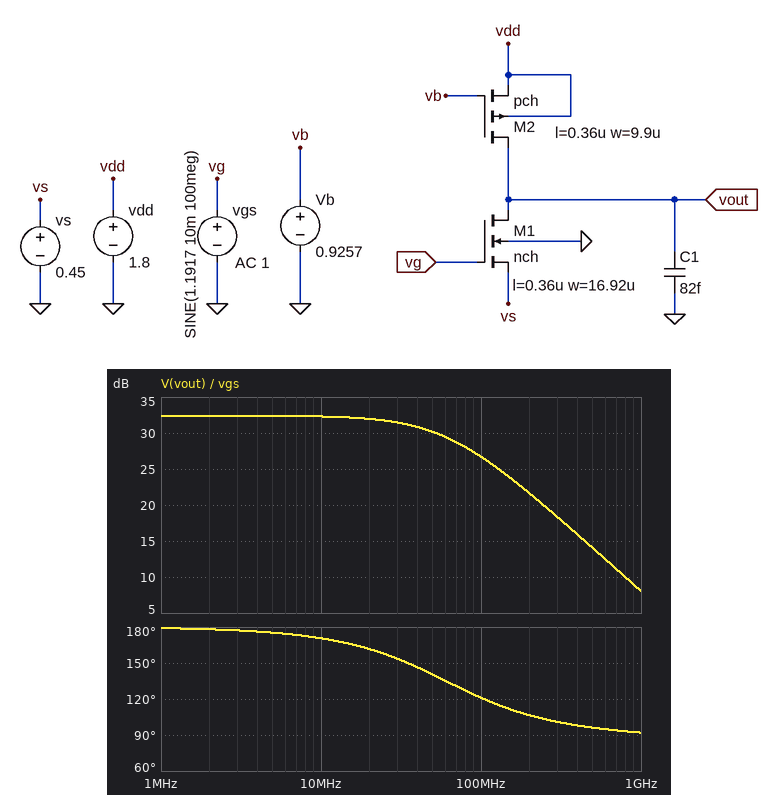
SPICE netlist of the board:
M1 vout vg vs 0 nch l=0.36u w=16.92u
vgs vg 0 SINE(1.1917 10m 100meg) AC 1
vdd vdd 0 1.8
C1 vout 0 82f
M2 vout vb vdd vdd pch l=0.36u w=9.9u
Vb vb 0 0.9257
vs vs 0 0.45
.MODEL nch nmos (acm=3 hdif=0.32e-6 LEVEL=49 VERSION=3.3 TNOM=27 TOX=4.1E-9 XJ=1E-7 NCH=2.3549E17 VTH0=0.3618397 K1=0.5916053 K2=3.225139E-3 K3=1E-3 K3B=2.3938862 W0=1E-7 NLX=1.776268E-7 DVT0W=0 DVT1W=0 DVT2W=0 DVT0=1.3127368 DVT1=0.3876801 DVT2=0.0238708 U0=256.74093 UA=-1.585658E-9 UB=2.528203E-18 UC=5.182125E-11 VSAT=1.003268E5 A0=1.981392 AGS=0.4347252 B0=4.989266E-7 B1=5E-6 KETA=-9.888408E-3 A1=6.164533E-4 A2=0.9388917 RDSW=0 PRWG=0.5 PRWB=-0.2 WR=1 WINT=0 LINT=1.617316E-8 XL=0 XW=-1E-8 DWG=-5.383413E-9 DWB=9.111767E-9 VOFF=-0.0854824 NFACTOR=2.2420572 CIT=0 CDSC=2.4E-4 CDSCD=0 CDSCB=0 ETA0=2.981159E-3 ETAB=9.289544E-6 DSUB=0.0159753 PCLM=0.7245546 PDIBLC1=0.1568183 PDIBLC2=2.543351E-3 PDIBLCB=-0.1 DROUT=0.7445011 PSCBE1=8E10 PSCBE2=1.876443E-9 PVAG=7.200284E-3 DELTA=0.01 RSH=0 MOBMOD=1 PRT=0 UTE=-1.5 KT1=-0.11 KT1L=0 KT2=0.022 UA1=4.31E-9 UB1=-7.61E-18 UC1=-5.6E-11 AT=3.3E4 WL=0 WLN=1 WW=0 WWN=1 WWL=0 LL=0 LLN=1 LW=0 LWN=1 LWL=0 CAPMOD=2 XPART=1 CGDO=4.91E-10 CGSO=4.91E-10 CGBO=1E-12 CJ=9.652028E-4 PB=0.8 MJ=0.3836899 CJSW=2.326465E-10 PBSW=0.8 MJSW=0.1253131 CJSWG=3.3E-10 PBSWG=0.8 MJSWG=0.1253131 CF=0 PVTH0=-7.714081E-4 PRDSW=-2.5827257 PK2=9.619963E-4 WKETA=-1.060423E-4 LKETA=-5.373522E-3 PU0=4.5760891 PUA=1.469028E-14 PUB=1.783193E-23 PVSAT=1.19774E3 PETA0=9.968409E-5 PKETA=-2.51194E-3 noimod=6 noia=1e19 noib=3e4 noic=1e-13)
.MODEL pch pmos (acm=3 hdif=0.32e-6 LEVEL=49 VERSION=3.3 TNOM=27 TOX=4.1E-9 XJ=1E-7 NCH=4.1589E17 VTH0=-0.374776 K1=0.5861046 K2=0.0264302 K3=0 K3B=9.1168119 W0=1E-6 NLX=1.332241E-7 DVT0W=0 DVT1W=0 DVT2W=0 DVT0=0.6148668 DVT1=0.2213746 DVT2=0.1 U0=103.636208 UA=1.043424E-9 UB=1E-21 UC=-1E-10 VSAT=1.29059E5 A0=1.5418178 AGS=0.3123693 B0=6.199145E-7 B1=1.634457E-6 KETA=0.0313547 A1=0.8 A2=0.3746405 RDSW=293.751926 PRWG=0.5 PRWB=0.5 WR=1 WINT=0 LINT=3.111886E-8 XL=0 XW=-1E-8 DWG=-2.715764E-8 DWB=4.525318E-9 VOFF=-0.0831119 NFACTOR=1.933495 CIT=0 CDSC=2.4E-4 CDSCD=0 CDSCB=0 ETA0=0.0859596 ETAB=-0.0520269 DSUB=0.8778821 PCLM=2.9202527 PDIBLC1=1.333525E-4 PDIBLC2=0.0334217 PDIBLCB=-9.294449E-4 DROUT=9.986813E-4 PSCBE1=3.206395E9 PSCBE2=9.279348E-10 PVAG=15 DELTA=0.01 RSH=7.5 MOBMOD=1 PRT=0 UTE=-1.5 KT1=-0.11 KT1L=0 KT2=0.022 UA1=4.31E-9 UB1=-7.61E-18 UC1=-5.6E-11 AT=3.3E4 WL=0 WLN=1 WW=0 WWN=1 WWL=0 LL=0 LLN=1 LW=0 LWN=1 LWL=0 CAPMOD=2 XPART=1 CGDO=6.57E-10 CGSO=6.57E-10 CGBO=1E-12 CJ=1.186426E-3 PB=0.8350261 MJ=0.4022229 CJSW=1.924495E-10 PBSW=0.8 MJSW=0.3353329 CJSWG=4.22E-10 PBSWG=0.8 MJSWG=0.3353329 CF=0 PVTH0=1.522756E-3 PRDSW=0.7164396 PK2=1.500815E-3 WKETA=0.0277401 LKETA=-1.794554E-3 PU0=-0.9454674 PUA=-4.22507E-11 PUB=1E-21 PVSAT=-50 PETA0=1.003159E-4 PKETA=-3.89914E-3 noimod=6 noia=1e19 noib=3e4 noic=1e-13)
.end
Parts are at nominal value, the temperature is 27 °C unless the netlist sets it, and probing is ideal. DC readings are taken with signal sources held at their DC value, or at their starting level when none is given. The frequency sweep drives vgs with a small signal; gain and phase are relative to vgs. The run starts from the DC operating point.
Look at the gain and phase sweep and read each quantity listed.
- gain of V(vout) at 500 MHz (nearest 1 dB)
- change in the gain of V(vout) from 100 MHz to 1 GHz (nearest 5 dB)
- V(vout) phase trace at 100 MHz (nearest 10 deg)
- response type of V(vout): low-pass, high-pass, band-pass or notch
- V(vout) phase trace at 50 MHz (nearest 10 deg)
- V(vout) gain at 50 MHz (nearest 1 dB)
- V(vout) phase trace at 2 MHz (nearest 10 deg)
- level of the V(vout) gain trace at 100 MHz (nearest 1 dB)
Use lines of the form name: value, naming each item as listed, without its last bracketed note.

gain of V(vout) at 500 MHz: 14 dB
change in the gain of V(vout) from 100 MHz to 1 GHz: -20 dB
V(vout) phase trace at 100 MHz: 120 deg
response type of V(vout): low-pass, high-pass, band-pass or notch: low-pass
V(vout) phase trace at 50 MHz: 140 deg
V(vout) gain at 50 MHz: 30 dB
V(vout) phase trace at 2 MHz: 180 deg
level of the V(vout) gain trace at 100 MHz: 27 dB
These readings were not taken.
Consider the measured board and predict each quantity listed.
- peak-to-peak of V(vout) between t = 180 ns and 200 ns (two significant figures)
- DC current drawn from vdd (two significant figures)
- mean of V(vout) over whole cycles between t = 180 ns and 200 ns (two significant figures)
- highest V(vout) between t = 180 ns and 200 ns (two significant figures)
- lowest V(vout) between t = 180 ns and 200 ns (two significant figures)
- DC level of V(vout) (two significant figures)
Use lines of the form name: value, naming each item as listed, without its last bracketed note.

peak-to-peak of V(vout) between t = 180 ns and 200 ns: 430 mV
DC current drawn from vdd: 170 µA
mean of V(vout) over whole cycles between t = 180 ns and 200 ns: 1.1 V
highest V(vout) between t = 180 ns and 200 ns: 1.3 V
lowest V(vout) between t = 180 ns and 200 ns: 880 mV
DC level of V(vout): 1.1 V
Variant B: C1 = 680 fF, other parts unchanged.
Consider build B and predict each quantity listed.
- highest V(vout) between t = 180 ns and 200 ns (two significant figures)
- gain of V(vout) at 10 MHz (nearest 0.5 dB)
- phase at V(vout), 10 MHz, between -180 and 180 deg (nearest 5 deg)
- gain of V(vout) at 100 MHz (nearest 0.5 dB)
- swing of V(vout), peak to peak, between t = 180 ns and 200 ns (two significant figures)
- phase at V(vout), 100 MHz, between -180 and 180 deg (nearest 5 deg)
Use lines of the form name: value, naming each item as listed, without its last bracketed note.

highest V(vout) between t = 180 ns and 200 ns: 1.1 V
gain of V(vout) at 10 MHz: 29.5 dB
phase at V(vout), 10 MHz, between -180 and 180 deg: 135 deg
gain of V(vout) at 100 MHz: 12.5 dB
swing of V(vout), peak to peak, between t = 180 ns and 200 ns: 86 mV
phase at V(vout), 100 MHz, between -180 and 180 deg: 95 deg
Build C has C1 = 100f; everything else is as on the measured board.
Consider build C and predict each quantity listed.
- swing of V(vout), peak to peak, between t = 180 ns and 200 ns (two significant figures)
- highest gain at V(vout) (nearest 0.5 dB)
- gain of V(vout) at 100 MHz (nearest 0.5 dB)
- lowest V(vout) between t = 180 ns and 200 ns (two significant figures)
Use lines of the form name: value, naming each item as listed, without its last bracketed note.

swing of V(vout), peak to peak, between t = 180 ns and 200 ns: 390 mV
highest gain at V(vout): 32.5 dB
gain of V(vout) at 100 MHz: 26.0 dB
lowest V(vout) between t = 180 ns and 200 ns: 900 mV
